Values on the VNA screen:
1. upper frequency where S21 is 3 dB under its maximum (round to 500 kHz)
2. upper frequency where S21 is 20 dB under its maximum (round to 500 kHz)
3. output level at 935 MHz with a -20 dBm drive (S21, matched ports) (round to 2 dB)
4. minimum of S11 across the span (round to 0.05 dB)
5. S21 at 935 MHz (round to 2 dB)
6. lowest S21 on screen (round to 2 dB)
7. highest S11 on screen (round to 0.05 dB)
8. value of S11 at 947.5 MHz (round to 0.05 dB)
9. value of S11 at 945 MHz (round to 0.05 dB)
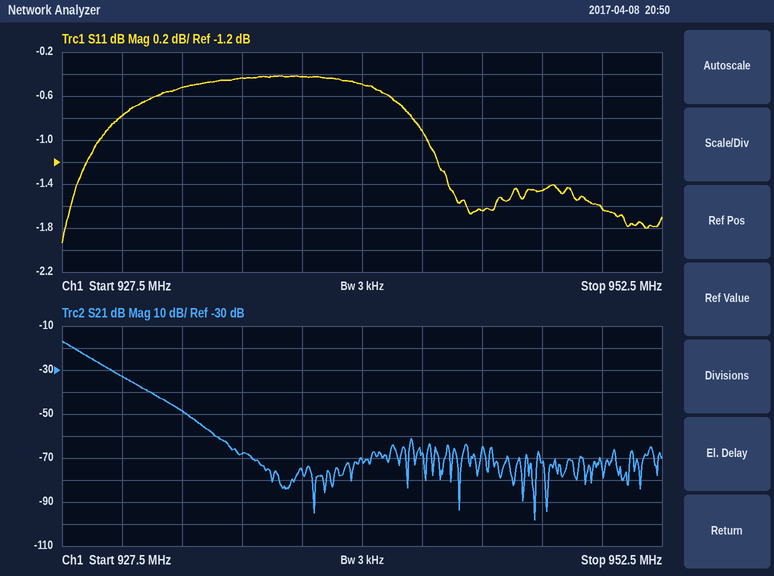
928.0 MHz
930.5 MHz
-88 dBm
-1.95 dB
-68 dB
-98 dB
-0.40 dB
-1.45 dB
-1.65 dB
